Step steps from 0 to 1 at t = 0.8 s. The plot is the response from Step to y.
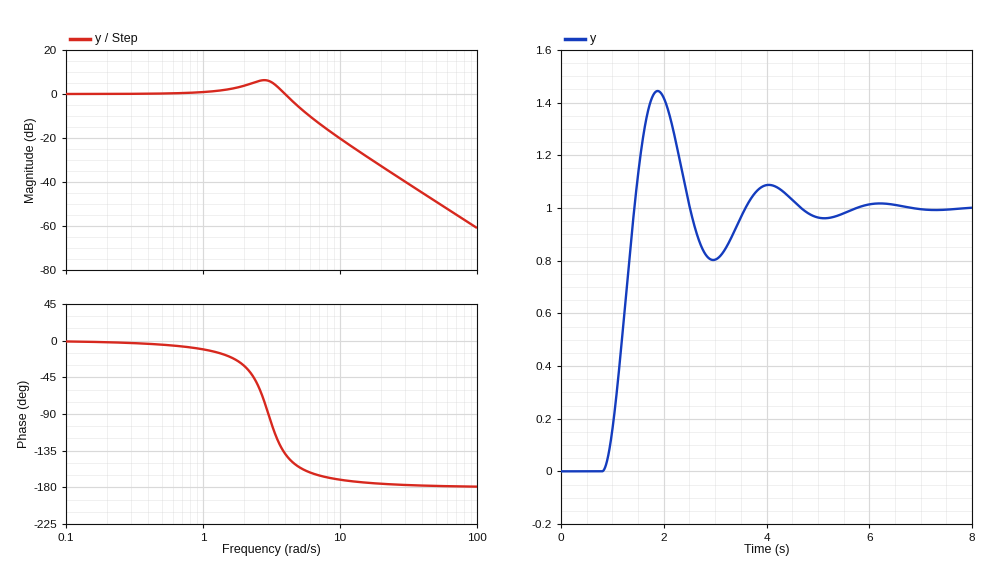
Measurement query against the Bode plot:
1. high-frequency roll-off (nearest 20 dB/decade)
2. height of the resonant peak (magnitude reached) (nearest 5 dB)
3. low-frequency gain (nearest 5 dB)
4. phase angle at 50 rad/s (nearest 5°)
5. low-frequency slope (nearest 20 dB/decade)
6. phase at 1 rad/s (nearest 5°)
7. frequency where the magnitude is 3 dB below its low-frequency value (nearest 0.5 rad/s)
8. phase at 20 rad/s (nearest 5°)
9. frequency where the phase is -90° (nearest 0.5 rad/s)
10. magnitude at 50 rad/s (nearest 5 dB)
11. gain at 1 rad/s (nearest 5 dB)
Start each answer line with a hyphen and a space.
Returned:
- -40 dB/decade
- 5 dB
- 0 dB
- -180°
- 0 dB/decade
- -10°
- 4.5 rad/s
- -175°
- 3.0 rad/s
- -50 dB
- 0 dB
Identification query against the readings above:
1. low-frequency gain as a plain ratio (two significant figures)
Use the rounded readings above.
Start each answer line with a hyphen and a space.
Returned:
- 1.0
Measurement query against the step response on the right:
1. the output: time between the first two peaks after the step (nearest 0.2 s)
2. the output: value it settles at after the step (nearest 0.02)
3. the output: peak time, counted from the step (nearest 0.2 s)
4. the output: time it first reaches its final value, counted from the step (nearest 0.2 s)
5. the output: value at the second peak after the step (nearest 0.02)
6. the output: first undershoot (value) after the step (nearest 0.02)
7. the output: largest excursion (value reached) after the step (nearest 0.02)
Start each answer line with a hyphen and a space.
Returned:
- 2.2 s
- 1.00
- 1.0 s
- 0.6 s
- 1.08
- 0.80
- 1.44
